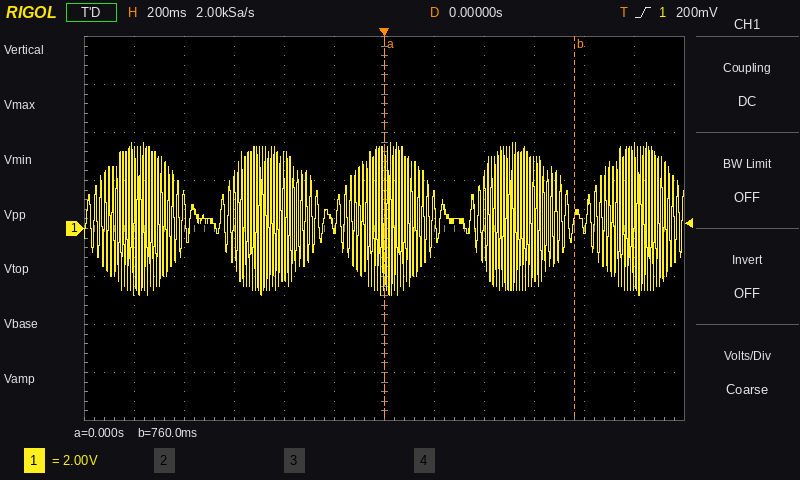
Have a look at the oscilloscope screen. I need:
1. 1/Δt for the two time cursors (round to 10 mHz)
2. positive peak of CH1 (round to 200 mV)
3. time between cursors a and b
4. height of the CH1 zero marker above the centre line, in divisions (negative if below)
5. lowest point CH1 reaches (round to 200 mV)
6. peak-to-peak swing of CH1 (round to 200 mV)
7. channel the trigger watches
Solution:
1.32 Hz
3.6 V
760 ms
0.0 div
-2.8 V
6.4 V
CH1
